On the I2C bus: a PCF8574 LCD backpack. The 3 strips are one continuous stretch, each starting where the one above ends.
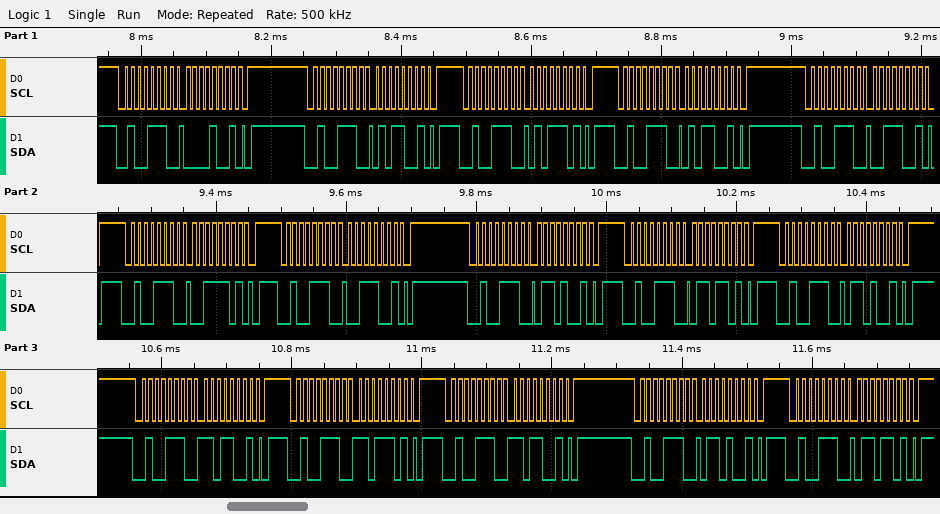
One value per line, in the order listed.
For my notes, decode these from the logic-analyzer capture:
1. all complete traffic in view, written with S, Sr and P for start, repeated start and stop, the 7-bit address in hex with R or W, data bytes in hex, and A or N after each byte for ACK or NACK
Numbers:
S 27W A 09 A P S 27W A 59 A P S 27W A 5D A P S 27W A 59 A P S 27W A 39 A P S 27W A 3D A P S 27W A 39 A P S 27W A 69 A P S 27W A 6D A P S 27W A 69 A P S 27W A D9 A P S 27W A DD A P S 27W A D9 A P S 27W A 69 A P S 27W A 6D A P
